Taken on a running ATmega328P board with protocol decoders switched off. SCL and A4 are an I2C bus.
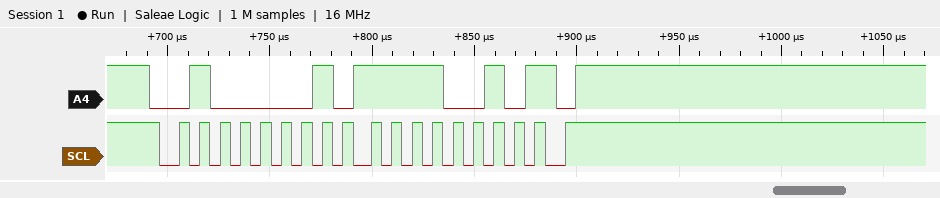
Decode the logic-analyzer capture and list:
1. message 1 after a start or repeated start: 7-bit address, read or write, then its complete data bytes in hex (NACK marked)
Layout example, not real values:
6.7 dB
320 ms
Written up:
0x20 read: F2 NACK
